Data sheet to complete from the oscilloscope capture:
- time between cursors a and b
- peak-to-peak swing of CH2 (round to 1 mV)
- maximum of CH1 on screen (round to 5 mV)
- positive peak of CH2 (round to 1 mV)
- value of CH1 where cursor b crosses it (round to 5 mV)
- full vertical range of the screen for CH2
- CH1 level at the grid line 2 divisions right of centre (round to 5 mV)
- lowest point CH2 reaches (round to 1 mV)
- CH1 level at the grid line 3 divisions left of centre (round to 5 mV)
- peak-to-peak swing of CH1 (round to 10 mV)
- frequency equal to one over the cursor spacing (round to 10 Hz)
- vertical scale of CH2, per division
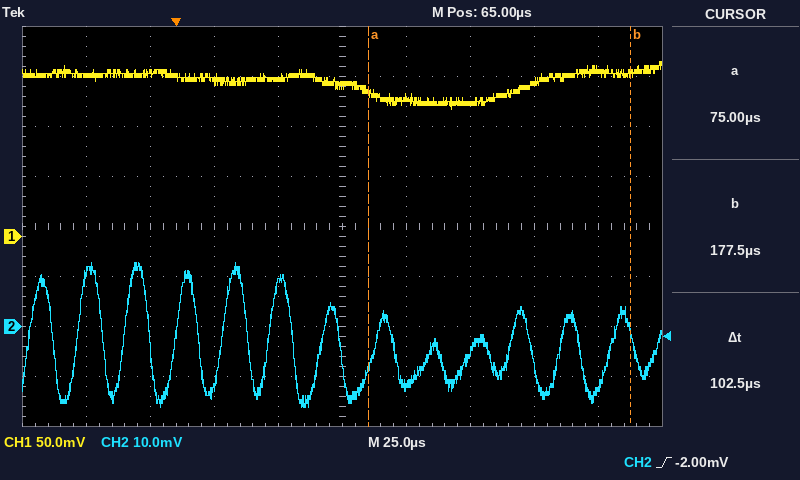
102.5 µs
29 mV
175 mV
13 mV
165 mV
80 mV
135 mV
-16 mV
165 mV
50 mV
9.76 kHz
10 mV
